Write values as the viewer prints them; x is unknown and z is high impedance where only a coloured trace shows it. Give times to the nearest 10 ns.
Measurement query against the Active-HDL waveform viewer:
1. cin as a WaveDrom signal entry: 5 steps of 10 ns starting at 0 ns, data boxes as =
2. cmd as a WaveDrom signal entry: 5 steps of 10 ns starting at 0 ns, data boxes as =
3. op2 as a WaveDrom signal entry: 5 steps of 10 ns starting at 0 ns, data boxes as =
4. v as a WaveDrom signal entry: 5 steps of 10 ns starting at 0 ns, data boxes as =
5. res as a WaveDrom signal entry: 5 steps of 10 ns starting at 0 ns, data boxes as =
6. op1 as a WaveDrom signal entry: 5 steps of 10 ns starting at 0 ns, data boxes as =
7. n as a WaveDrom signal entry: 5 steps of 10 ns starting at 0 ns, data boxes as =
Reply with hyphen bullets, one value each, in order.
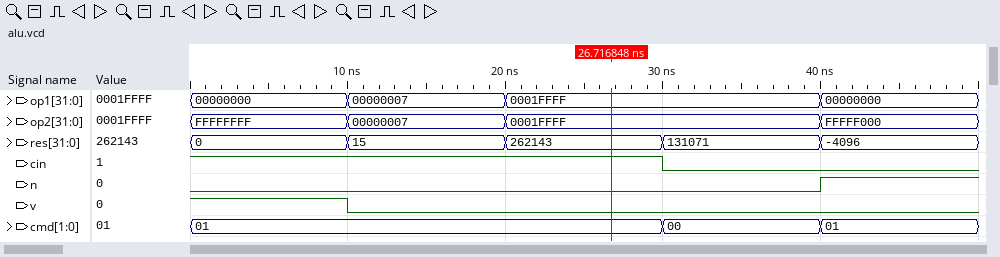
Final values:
- {name: 'cin', wave: '1..0.'}
- {name: 'cmd', wave: '=..==', data: '01 00 01'}
- {name: 'op2', wave: '===.=', data: 'FFFFFFFF 00000007 0001FFFF FFFFF000'}
- {name: 'v', wave: '10...'}
- {name: 'res', wave: '=====', data: '0 15 262143 131071 -4096'}
- {name: 'op1', wave: '===.=', data: '00000000 00000007 0001FFFF 00000000'}
- {name: 'n', wave: '0...1'}
